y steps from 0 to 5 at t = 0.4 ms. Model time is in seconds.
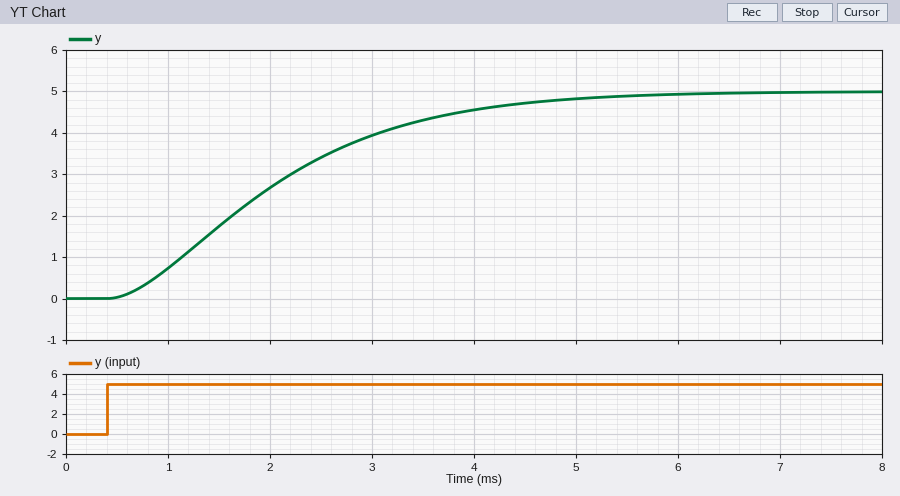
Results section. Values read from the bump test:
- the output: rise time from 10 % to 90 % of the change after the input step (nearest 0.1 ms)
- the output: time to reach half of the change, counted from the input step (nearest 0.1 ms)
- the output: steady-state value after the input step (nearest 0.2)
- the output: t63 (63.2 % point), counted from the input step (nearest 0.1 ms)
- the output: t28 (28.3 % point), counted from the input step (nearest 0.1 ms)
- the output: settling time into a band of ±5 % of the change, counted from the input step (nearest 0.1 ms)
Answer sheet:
3.0 ms
1.5 ms
5.0
1.9 ms
0.9 ms
4.2 ms
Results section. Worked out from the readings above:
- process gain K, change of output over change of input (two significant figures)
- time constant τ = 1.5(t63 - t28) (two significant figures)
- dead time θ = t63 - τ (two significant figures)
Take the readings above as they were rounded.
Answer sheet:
1.0
1.5 ms
0.40 ms
